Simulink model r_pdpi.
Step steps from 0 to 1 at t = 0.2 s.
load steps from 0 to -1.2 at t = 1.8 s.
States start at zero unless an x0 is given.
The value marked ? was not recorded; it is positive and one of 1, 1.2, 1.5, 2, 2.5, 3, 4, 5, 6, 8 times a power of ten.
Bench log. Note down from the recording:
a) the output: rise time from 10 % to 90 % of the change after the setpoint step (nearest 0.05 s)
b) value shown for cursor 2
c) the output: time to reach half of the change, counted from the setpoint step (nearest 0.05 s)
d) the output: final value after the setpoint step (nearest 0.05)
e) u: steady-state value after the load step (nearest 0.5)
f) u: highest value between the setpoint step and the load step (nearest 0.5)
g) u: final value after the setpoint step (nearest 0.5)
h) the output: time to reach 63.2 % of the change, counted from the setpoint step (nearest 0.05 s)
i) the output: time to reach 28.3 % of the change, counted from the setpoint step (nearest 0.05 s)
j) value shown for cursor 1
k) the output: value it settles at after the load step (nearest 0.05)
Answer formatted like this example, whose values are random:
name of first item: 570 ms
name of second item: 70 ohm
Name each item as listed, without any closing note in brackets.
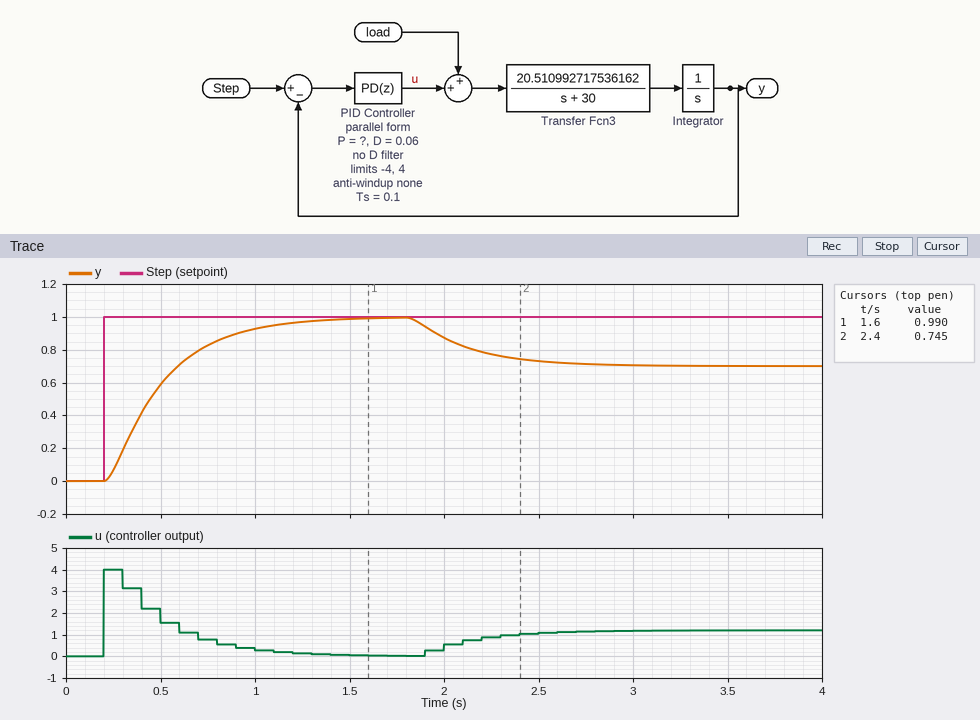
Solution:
the output: rise time from 10 % to 90 % of the change after the setpoint step: 0.65 s
value shown for cursor 2: 0.745
the output: time to reach half of the change, counted from the setpoint step: 0.25 s
the output: final value after the setpoint step: 1.00
u: steady-state value after the load step: 1.0
u: highest value between the setpoint step and the load step: 4.0
u: final value after the setpoint step: 0.0
the output: time to reach 63.2 % of the change, counted from the setpoint step: 0.35 s
the output: time to reach 28.3 % of the change, counted from the setpoint step: 0.15 s
value shown for cursor 1: 0.990
the output: value it settles at after the load step: 0.70
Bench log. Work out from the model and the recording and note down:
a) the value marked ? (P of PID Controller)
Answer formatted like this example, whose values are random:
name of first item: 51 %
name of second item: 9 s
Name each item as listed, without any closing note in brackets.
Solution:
the value marked ?: 4
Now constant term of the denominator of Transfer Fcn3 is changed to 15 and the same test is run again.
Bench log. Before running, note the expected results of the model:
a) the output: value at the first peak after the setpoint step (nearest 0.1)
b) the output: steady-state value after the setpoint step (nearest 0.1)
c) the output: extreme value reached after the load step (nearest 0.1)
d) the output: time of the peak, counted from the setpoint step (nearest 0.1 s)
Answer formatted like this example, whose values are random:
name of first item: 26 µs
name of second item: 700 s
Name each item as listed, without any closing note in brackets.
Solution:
the output: value at the first peak after the setpoint step: 1.1
the output: steady-state value after the setpoint step: 1.0
the output: extreme value reached after the load step: 0.7
the output: time of the peak, counted from the setpoint step: 0.5 s
